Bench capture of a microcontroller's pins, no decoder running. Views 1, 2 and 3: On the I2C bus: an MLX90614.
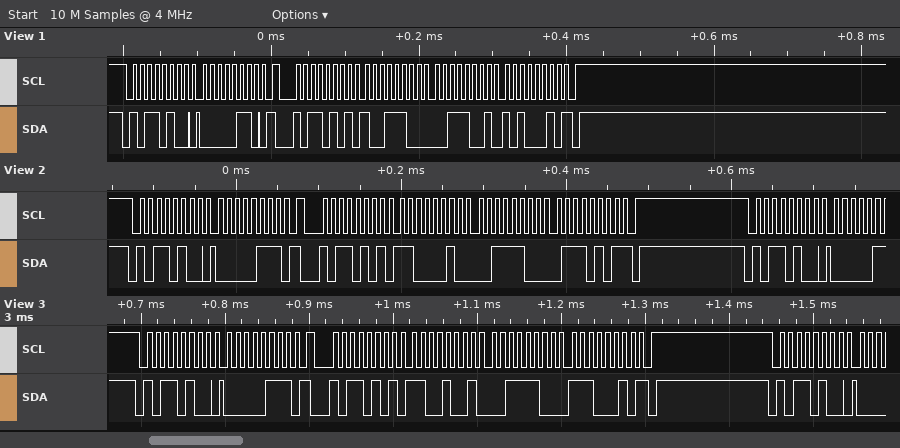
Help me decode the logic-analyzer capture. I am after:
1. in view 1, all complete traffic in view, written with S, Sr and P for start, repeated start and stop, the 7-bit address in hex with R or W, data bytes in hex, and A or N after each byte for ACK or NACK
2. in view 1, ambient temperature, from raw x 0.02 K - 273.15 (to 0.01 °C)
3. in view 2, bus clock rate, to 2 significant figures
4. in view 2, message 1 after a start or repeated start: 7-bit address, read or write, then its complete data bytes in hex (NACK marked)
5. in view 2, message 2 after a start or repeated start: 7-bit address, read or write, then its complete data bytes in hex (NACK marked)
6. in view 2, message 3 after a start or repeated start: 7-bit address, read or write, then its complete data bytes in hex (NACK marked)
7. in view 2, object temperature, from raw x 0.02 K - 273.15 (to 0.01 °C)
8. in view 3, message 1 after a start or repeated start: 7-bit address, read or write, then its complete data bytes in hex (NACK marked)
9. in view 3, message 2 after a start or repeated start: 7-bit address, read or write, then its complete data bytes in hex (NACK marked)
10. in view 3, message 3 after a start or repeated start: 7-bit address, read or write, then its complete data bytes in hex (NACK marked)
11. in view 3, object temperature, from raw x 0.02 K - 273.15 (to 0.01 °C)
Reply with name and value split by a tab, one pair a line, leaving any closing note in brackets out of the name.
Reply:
in view 1, all complete traffic in view, written with S, Sr and P for start, repeated start and stop, the 7-bit address in hex with R or W, data bytes in hex, and A or N after each byte for ACK or NACK	S 5AW A 06 A Sr 5AR A 9C A 39 A A2 N P
in view 1, ambient temperature, from raw x 0.02 K - 273.15	21.81 °C
in view 2, bus clock rate, to 2 significant figures	100 kHz
in view 2, message 1 after a start or repeated start: 7-bit address, read or write, then its complete data bytes in hex	0x5A write: 07
in view 2, message 2 after a start or repeated start: 7-bit address, read or write, then its complete data bytes in hex	0x5A read: C2 3C 75 NACK
in view 2, message 3 after a start or repeated start: 7-bit address, read or write, then its complete data bytes in hex	0x5A write
in view 2, object temperature, from raw x 0.02 K - 273.15	37.93 °C
in view 3, message 1 after a start or repeated start: 7-bit address, read or write, then its complete data bytes in hex	0x5A write: 07
in view 3, message 2 after a start or repeated start: 7-bit address, read or write, then its complete data bytes in hex	0x5A read: C9 3C E2 NACK
in view 3, message 3 after a start or repeated start: 7-bit address, read or write, then its complete data bytes in hex	0x5A write
in view 3, object temperature, from raw x 0.02 K - 273.15	38.07 °C
